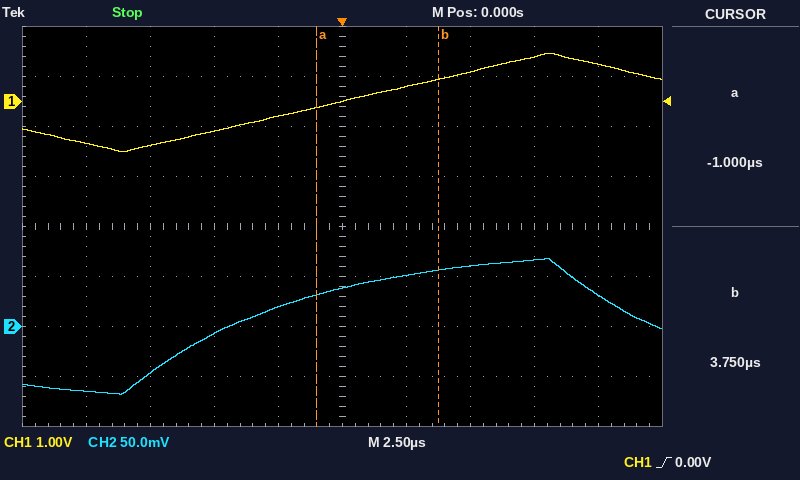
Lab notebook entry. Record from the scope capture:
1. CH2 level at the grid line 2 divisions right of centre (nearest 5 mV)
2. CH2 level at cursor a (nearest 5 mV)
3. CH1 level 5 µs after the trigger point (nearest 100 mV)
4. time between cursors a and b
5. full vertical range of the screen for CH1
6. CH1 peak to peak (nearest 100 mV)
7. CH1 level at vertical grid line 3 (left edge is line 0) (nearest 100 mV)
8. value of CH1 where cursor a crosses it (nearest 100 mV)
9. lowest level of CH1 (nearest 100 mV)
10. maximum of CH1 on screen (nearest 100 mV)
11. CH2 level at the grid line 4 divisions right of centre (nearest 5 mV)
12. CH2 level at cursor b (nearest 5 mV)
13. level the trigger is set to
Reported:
60 mV
30 mV
600 mV
4.75 µs
8 V
2.0 V
-600 mV
-100 mV
-1.0 V
1.0 V
30 mV
55 mV
0.00 V
